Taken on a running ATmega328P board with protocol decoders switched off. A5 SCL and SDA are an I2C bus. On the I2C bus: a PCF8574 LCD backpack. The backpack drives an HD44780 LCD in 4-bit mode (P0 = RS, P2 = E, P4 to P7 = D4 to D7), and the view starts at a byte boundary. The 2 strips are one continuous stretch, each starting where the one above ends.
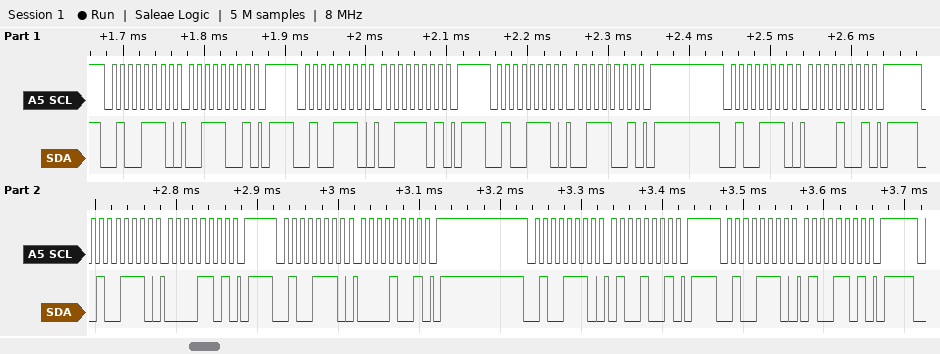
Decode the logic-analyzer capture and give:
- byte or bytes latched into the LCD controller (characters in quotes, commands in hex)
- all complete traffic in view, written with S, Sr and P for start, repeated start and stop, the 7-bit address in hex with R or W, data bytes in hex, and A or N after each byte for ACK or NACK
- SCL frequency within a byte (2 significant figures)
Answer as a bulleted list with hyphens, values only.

- '0'
- S 27W A 39 A P S 27W A 3D A P S 27W A 39 A P S 27W A 09 A P S 27W A 0D A P S 27W A 09 A P S 27W A 49 A P S 27W A 4D A P
- 100 kHz
